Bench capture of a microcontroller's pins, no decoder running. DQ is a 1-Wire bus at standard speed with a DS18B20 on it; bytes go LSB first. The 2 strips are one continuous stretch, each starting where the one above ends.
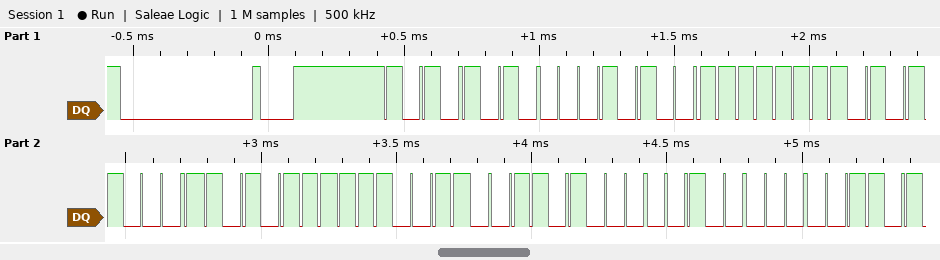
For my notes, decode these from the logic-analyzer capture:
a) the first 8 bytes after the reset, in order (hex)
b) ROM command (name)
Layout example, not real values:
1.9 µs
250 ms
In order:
55 28 FF 1A EB 67 16 04
Match ROM
